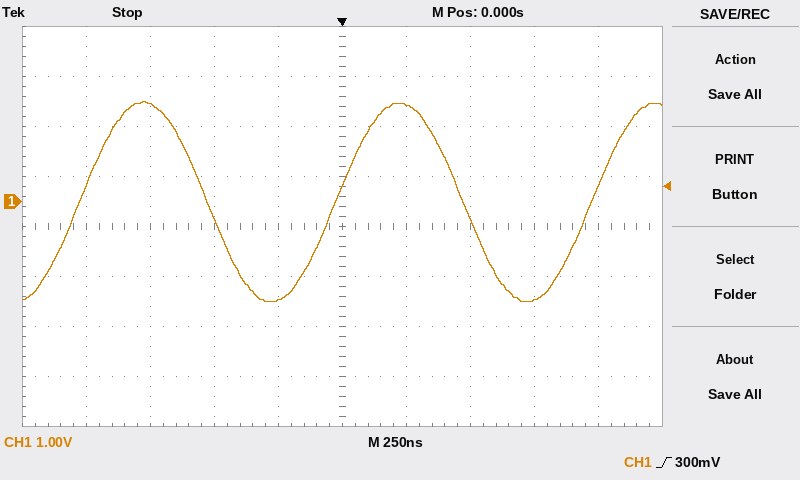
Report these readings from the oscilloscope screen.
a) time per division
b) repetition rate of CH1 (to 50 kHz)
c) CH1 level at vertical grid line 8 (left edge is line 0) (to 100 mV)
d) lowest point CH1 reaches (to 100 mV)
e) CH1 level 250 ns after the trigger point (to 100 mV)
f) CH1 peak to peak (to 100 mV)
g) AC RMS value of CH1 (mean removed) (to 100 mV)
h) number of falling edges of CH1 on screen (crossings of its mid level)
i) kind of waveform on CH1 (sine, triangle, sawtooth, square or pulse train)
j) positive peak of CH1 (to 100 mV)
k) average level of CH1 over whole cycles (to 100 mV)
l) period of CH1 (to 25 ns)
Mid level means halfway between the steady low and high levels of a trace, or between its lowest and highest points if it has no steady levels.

250 ns
1.00 MHz
-2.0 V
-2.0 V
1.9 V
4.0 V
1.4 V
2
sine
2.0 V
0.0 V
1.000 µs
